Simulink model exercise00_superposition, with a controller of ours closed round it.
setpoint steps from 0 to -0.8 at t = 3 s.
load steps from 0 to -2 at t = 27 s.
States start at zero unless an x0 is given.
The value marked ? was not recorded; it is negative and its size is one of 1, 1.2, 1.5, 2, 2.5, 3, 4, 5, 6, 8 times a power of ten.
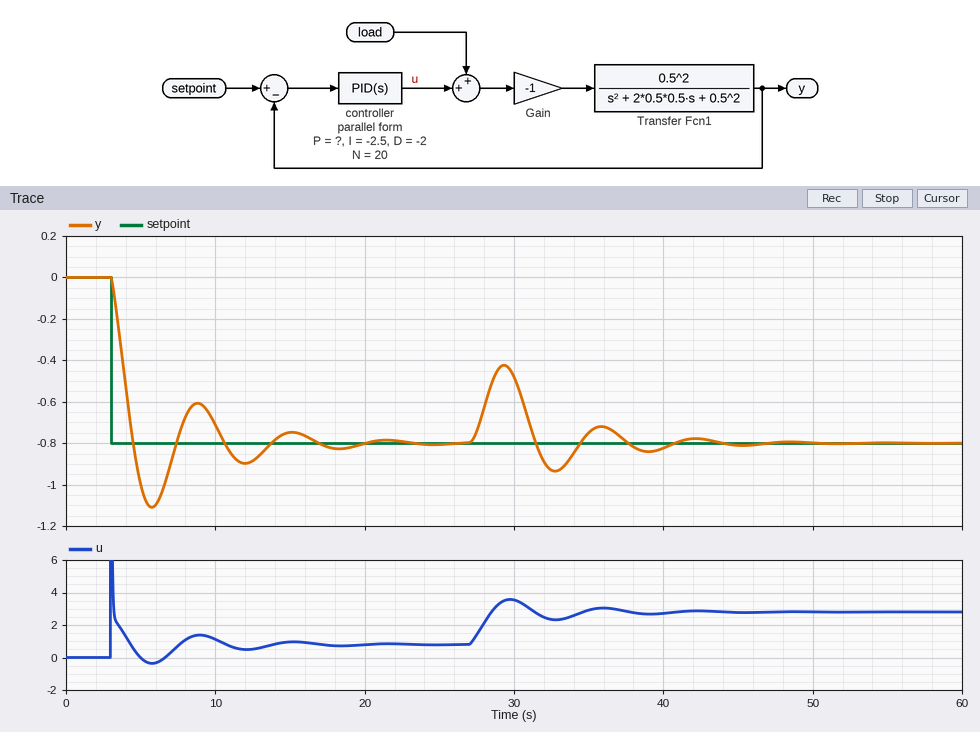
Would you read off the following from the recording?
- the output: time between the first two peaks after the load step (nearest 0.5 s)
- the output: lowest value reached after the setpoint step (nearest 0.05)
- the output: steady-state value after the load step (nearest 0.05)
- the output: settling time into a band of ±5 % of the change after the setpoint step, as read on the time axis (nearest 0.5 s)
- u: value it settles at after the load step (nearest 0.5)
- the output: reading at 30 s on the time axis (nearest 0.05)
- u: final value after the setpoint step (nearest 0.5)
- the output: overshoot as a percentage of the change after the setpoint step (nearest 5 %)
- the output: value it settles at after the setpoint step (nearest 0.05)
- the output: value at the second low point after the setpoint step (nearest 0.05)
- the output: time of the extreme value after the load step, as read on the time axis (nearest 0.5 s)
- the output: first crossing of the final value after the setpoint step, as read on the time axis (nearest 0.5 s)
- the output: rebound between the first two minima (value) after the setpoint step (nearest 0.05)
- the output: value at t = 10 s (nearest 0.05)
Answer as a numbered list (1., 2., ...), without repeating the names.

1. 6.5 s
2. -1.10
3. -0.80
4. 16.0 s
5. 3.0
6. -0.50
7. 1.0
8. 40 %
9. -0.80
10. -0.90
11. 29.5 s
12. 4.5 s
13. -0.60
14. -0.70
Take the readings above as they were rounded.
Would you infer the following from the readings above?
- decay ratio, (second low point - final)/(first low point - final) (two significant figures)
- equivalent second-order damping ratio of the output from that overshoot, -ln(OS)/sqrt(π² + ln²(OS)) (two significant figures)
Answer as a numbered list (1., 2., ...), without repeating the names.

1. 0.33
2. 0.28
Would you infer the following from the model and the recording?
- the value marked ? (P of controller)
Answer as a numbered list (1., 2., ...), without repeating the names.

1. -4
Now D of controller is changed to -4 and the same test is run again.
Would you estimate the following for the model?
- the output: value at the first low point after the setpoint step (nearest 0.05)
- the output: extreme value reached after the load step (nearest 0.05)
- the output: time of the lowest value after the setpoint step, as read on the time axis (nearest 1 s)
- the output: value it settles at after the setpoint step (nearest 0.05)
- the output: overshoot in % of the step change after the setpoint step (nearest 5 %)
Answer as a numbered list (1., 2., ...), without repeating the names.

1. -0.95
2. -0.50
3. 6 s
4. -0.80
5. 20 %
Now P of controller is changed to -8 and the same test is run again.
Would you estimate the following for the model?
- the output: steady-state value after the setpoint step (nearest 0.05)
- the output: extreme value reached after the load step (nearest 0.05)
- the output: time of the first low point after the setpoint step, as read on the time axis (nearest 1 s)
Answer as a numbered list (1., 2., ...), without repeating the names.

1. -0.80
2. -0.55
3. 5 s
